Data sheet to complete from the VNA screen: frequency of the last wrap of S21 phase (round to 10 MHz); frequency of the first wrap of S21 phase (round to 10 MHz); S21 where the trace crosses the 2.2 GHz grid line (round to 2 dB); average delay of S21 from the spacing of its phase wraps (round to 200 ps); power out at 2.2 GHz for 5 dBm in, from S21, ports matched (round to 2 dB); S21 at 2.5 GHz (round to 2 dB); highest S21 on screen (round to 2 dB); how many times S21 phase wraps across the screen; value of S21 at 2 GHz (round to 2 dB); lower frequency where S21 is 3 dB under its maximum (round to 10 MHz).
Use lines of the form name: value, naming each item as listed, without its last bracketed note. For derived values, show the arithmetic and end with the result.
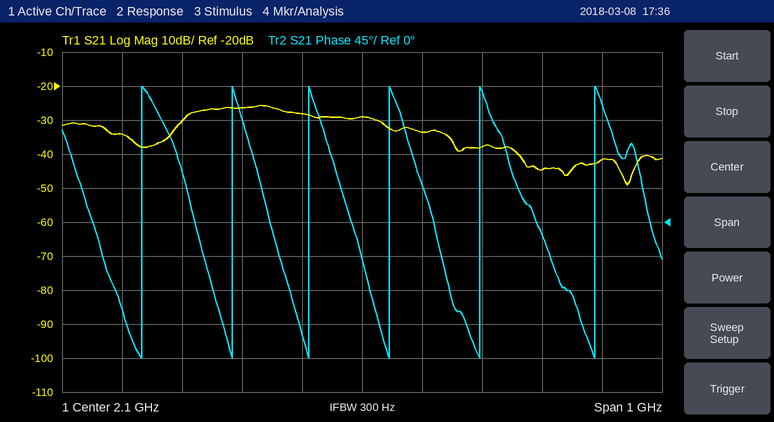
frequency of the last wrap of S21 phase: 2.49 GHz
frequency of the first wrap of S21 phase: 1.73 GHz
S21 where the trace crosses the 2.2 GHz grid line: -34 dB
average delay of S21 from the spacing of its phase wraps: 5 cycles / (2.49 GHz − 1.73 GHz) ≈ 6.6 ns
power out at 2.2 GHz for 5 dBm in, from S21, ports matched: 5 dBm + (-34 dB) = -28 dBm
S21 at 2.5 GHz: -42 dB
highest S21 on screen: -26 dB
how many times S21 phase wraps across the screen: 6
value of S21 at 2 GHz: -28 dB
lower frequency where S21 is 3 dB under its maximum: 1.81 GHz
